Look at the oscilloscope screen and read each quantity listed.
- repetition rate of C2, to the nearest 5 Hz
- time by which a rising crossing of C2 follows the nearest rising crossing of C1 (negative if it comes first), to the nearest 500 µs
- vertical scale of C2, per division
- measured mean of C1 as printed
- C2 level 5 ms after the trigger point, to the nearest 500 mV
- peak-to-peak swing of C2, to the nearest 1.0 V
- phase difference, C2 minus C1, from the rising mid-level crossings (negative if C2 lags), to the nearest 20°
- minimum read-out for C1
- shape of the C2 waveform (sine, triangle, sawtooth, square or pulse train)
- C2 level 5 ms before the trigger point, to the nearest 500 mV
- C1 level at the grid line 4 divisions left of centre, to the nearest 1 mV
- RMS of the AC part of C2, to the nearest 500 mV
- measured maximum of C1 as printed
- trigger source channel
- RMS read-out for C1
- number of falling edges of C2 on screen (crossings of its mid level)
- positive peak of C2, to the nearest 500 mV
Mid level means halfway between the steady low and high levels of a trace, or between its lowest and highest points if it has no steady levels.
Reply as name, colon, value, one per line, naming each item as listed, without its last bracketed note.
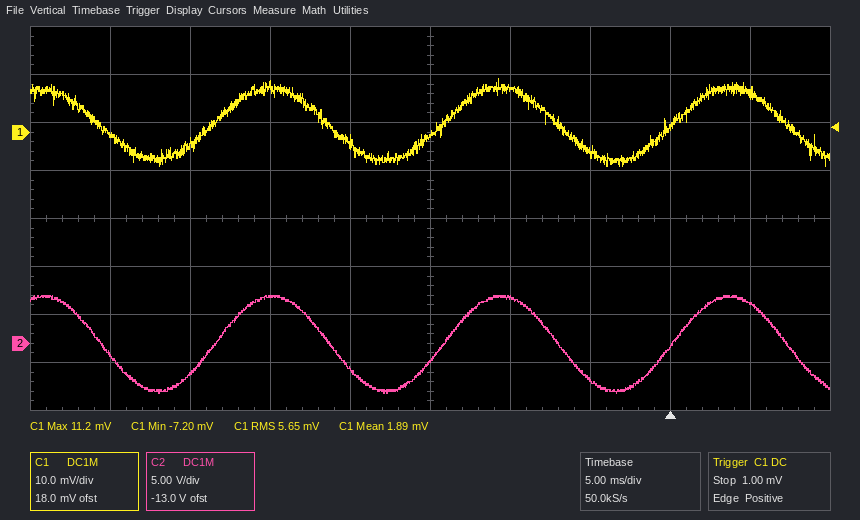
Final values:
repetition rate of C2, to the nearest 5 Hz: 70 Hz
time by which a rising crossing of C2 follows the nearest rising crossing of C1 (negative if it comes first), to the nearest 500 µs: 0.0 ms
vertical scale of C2, per division: 5 V
measured mean of C1 as printed: 1.89 mV
C2 level 5 ms after the trigger point, to the nearest 500 mV: 4.0 V
peak-to-peak swing of C2, to the nearest 1.0 V: 10.0 V
phase difference, C2 minus C1, from the rising mid-level crossings (negative if C2 lags), to the nearest 20°: 0°
minimum read-out for C1: -7.20 mV
shape of the C2 waveform: sine
C2 level 5 ms before the trigger point, to the nearest 500 mV: -4.0 V
C1 level at the grid line 4 divisions left of centre, to the nearest 1 mV: 0 mV
RMS of the AC part of C2, to the nearest 500 mV: 3.5 V
measured maximum of C1 as printed: 11.2 mV
trigger source channel: C1
RMS read-out for C1: 5.65 mV
number of falling edges of C2 on screen: 4
positive peak of C2, to the nearest 500 mV: 5.0 V
